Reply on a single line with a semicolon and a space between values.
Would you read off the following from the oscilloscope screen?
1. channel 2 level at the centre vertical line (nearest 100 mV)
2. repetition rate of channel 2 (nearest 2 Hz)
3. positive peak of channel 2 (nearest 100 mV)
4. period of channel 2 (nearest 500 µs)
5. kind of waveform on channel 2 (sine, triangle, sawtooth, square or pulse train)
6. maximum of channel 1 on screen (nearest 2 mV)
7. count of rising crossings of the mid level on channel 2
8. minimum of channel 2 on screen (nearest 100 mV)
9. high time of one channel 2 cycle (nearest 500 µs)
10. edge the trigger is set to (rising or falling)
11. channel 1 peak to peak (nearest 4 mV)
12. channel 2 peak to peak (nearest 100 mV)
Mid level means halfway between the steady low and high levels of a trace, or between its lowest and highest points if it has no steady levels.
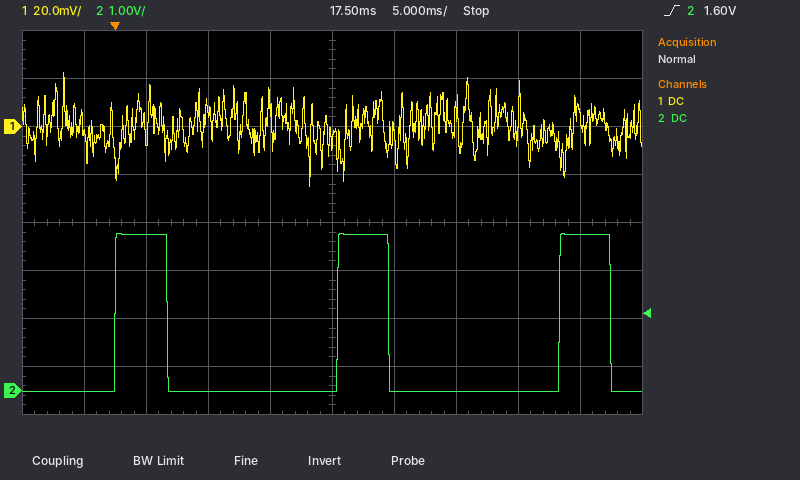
0.0 V; 56 Hz; 3.3 V; 18.0 ms; pulse train; 22 mV; 3; 0.0 V; 4.0 ms; rising; 48 mV; 3.3 V
